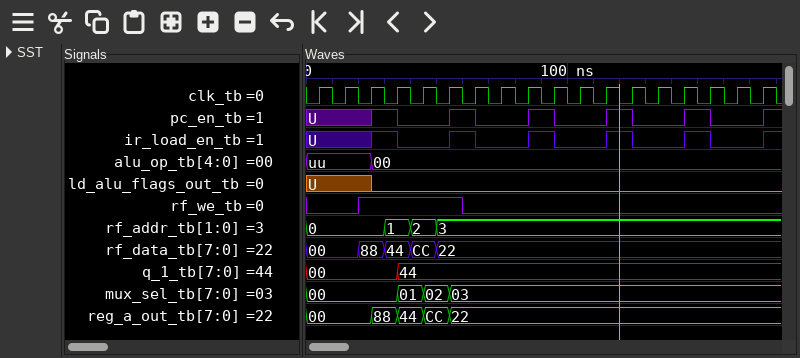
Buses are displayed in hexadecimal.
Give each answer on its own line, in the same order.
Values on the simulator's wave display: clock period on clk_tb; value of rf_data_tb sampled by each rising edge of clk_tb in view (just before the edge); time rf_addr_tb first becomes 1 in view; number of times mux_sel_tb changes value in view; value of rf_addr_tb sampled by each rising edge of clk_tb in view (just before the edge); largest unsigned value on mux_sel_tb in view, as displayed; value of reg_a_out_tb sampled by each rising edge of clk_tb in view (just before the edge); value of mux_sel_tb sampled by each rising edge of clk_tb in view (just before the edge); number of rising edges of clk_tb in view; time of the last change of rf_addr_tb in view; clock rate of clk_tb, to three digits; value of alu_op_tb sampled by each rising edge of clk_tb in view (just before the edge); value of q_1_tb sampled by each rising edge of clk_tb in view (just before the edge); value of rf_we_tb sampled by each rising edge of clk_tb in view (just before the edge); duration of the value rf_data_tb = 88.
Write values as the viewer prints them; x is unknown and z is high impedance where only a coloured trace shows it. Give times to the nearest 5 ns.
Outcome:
10 ns
00, 00, 88, 44, CC, 22, 22, 22, 22, 22, 22, 22, 22, 22, 22, 22, 22, 22
30 ns
3
0, 0, 0, 1, 2, 3, 3, 3, 3, 3, 3, 3, 3, 3, 3, 3, 3, 3
03
00, 00, 00, 88, 44, CC, 22, 22, 22, 22, 22, 22, 22, 22, 22, 22, 22, 22
00, 00, 00, 00, 01, 02, 03, 03, 03, 03, 03, 03, 03, 03, 03, 03, 03, 03
18
50 ns
100 MHz
uu, uu, uu, 00, 00, 00, 00, 00, 00, 00, 00, 00, 00, 00, 00, 00, 00, 00
00, 00, 00, 00, 44, 44, 44, 44, 44, 44, 44, 44, 44, 44, 44, 44, 44, 44
0 0 1 1 1 1 0 0 0 0 0 0 0 0 0 0 0 0
10 ns
